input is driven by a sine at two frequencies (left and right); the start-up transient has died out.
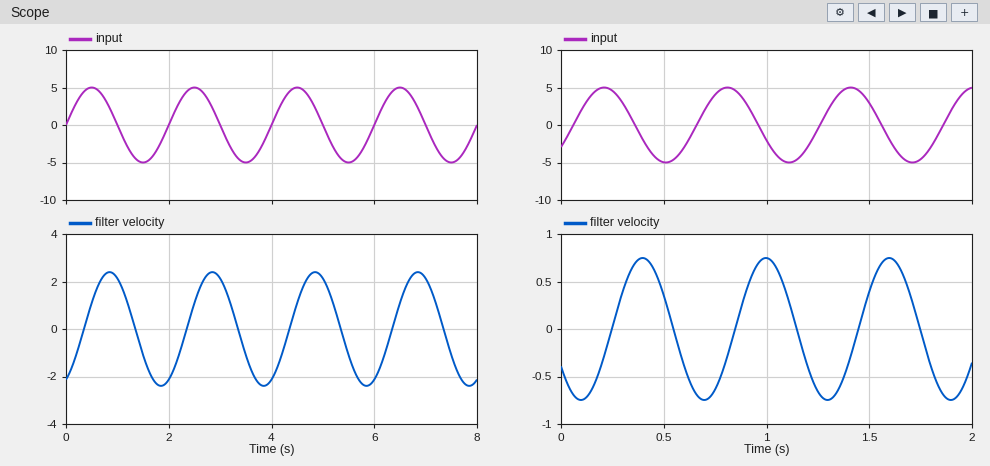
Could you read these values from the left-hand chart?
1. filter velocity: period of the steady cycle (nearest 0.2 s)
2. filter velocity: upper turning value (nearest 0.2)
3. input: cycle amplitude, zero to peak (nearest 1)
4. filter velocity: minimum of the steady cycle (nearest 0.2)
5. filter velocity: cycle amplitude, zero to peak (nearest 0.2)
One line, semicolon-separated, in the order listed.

2.0 s; 2.4; 5; -2.4; 2.4
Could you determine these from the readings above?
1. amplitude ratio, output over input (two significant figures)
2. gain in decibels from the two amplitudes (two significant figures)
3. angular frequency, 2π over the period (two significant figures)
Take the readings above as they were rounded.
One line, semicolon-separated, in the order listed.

0.48; -6.4 dB; 3.1 rad/s
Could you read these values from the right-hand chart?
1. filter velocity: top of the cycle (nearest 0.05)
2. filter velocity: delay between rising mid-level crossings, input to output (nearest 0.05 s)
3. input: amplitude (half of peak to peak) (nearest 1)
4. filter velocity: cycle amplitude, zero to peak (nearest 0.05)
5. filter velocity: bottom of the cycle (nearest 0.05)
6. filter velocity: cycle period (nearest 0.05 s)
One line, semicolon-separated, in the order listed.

0.75; 0.20 s; 5; 0.75; -0.75; 0.60 s
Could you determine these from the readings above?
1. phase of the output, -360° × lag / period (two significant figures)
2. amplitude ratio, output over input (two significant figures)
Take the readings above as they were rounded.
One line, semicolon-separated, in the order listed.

-120°; 0.15
